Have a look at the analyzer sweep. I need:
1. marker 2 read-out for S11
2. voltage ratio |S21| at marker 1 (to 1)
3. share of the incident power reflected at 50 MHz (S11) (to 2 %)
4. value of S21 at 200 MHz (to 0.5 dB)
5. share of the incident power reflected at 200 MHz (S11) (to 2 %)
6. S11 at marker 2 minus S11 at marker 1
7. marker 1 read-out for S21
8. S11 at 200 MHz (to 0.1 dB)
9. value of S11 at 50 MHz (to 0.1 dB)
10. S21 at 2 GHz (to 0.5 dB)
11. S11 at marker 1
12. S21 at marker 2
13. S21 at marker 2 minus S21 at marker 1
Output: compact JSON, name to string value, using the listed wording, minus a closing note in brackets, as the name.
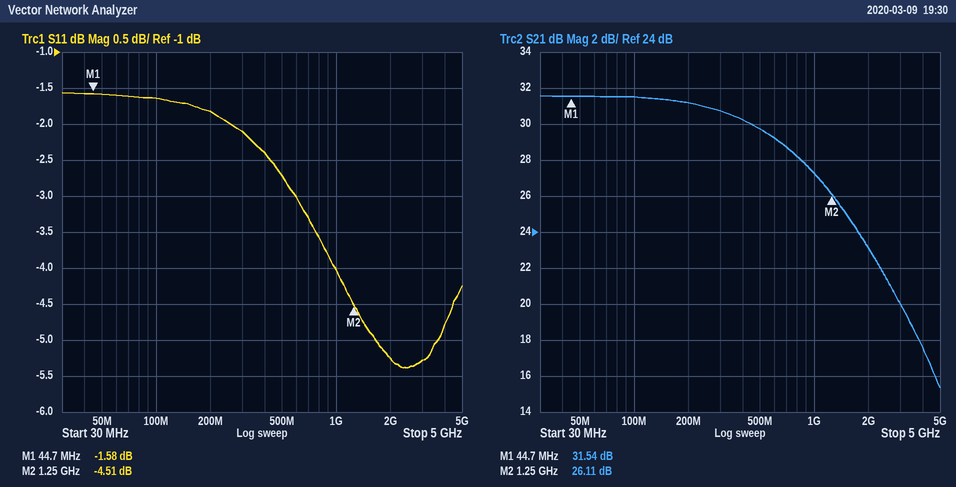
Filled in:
{"marker 2 read-out for S11": "-4.51 dB", "voltage ratio |S21| at marker 1": "38", "share of the incident power reflected at 50 MHz (S11)": "70 %", "value of S21 at 200 MHz": "31.0 dB", "share of the incident power reflected at 200 MHz (S11)": "66 %", "S11 at marker 2 minus S11 at marker 1": "-2.93 dB", "marker 1 read-out for S21": "31.54 dB", "S11 at 200 MHz": "-1.8 dB", "value of S11 at 50 MHz": "-1.6 dB", "S21 at 2 GHz": "23.0 dB", "S11 at marker 1": "-1.58 dB", "S21 at marker 2": "26.11 dB", "S21 at marker 2 minus S21 at marker 1": "-5.43 dB"}
